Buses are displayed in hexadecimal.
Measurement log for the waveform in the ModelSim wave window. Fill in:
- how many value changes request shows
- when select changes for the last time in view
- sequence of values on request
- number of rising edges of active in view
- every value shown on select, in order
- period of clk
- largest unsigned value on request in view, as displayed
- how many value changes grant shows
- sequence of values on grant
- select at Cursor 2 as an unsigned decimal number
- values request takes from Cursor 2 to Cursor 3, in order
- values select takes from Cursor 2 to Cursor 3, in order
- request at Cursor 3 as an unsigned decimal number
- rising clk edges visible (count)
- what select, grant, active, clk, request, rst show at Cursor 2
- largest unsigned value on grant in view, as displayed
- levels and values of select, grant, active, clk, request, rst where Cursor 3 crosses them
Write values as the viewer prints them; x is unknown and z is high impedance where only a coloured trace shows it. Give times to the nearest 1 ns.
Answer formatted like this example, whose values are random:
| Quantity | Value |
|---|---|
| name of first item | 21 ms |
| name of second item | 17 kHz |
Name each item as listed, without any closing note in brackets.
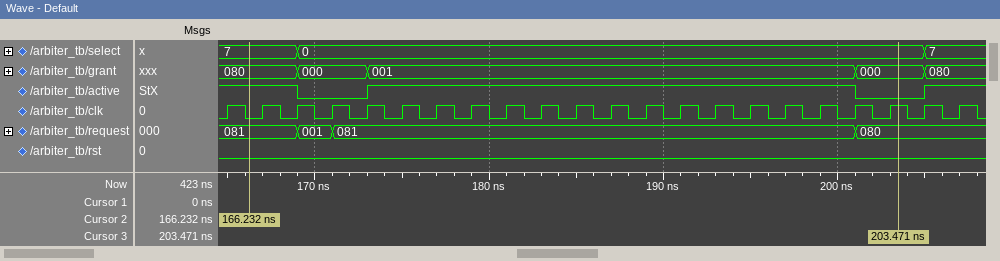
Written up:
| Quantity | Value |
|---|---|
| how many value changes request shows | 3 |
| when select changes for the last time in view | 205 ns |
| sequence of values on request | 081, 001, 081, 080 |
| number of rising edges of active in view | 2 |
| every value shown on select, in order | 7, 0, 7 |
| period of clk | 2 ns |
| largest unsigned value on request in view, as displayed | 081 |
| how many value changes grant shows | 4 |
| sequence of values on grant | 080, 000, 001, 000, 080 |
| select at Cursor 2 as an unsigned decimal number | 7 |
| values request takes from Cursor 2 to Cursor 3, in order | 081, 001, 081, 080 |
| values select takes from Cursor 2 to Cursor 3, in order | 7, 0 |
| request at Cursor 3 as an unsigned decimal number | 128 |
| rising clk edges visible | 22 |
| what select, grant, active, clk, request, rst show at Cursor 2 | select=7, grant=080, active=1, clk=0, request=081, rst=0 |
| largest unsigned value on grant in view, as displayed | 080 |
| levels and values of select, grant, active, clk, request, rst where Cursor 3 crosses them | select=0, grant=000, active=0, clk=1, request=080, rst=0 |
